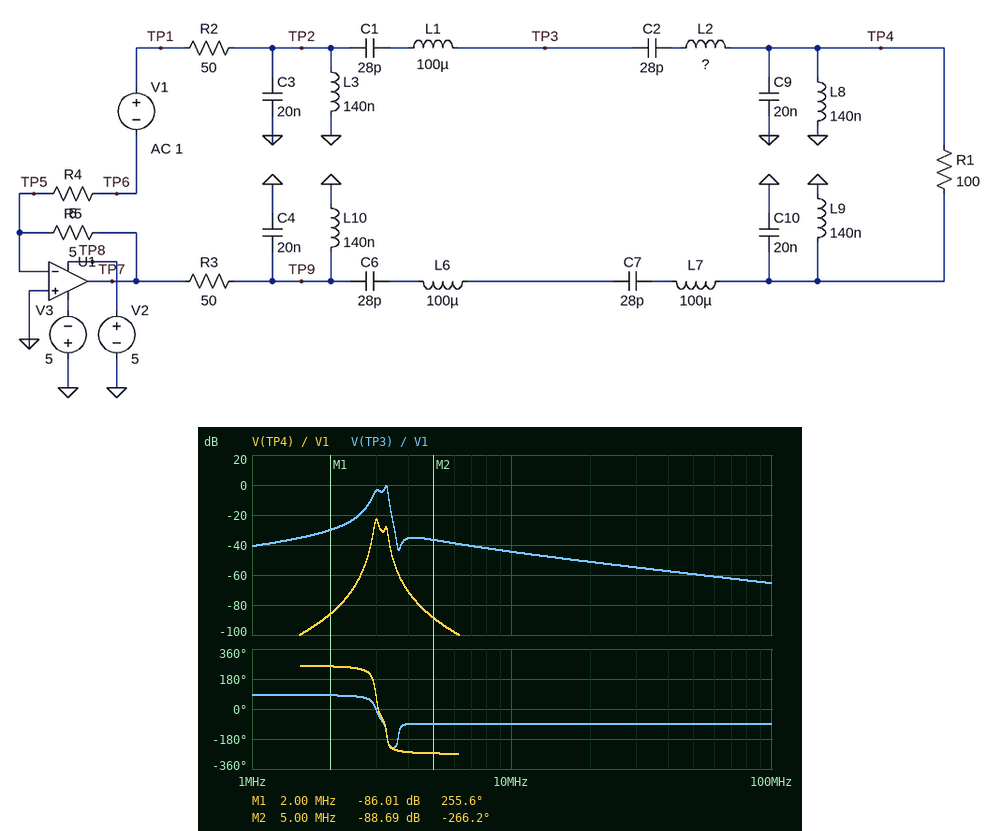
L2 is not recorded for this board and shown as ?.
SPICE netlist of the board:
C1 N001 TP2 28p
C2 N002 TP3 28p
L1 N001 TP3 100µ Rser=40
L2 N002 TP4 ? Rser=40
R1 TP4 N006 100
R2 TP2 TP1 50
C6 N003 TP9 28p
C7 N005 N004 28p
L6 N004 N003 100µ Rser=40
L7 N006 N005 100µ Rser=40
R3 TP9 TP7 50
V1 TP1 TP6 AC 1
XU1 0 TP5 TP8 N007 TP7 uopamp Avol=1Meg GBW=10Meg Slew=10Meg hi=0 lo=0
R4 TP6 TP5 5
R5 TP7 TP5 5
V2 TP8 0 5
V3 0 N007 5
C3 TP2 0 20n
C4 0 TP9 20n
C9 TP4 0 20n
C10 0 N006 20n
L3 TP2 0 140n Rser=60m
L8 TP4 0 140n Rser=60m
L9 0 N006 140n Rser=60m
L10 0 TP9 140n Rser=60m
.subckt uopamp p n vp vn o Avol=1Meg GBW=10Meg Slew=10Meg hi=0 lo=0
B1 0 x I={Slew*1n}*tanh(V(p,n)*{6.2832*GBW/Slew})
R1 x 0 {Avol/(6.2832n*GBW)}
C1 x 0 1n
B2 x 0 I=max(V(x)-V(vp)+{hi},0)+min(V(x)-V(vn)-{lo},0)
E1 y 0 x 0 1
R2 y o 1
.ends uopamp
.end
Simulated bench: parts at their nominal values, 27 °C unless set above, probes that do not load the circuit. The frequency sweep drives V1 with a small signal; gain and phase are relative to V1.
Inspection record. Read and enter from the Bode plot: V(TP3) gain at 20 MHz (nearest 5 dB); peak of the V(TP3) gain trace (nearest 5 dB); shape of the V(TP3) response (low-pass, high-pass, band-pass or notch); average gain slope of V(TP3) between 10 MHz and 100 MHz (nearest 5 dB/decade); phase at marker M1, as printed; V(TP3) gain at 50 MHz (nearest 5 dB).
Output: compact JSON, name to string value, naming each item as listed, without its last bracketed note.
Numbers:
{"V(TP3) gain at 20 MHz": "-50 dB", "peak of the V(TP3) gain trace": "0 dB", "shape of the V(TP3) response": "band-pass", "average gain slope of V(TP3) between 10 MHz and 100 MHz": "-20 dB/decade", "phase at marker M1, as printed": "255.6 deg", "V(TP3) gain at 50 MHz": "-60 dB"}
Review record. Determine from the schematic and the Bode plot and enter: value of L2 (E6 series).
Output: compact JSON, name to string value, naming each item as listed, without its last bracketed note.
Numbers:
{"value of L2": "68 µH"}
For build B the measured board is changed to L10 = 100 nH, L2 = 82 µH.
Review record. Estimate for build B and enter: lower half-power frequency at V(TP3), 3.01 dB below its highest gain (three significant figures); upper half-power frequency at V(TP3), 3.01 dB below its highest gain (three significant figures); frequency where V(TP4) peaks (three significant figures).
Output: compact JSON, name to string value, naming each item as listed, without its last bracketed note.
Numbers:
{"lower half-power frequency at V(TP3), 3.01 dB below its highest gain": "2.97 MHz", "upper half-power frequency at V(TP3), 3.01 dB below its highest gain": "3.19 MHz", "frequency where V(TP4) peaks": "3.02 MHz"}
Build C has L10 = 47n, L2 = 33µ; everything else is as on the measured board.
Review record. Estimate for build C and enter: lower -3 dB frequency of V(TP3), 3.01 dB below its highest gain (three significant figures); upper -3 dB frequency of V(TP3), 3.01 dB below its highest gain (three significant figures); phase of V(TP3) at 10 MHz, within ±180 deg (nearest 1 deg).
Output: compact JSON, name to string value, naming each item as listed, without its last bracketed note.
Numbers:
{"lower -3 dB frequency of V(TP3), 3.01 dB below its highest gain": "3.64 MHz", "upper -3 dB frequency of V(TP3), 3.01 dB below its highest gain": "3.74 MHz", "phase of V(TP3) at 10 MHz, within ±180 deg": "-93 deg"}
